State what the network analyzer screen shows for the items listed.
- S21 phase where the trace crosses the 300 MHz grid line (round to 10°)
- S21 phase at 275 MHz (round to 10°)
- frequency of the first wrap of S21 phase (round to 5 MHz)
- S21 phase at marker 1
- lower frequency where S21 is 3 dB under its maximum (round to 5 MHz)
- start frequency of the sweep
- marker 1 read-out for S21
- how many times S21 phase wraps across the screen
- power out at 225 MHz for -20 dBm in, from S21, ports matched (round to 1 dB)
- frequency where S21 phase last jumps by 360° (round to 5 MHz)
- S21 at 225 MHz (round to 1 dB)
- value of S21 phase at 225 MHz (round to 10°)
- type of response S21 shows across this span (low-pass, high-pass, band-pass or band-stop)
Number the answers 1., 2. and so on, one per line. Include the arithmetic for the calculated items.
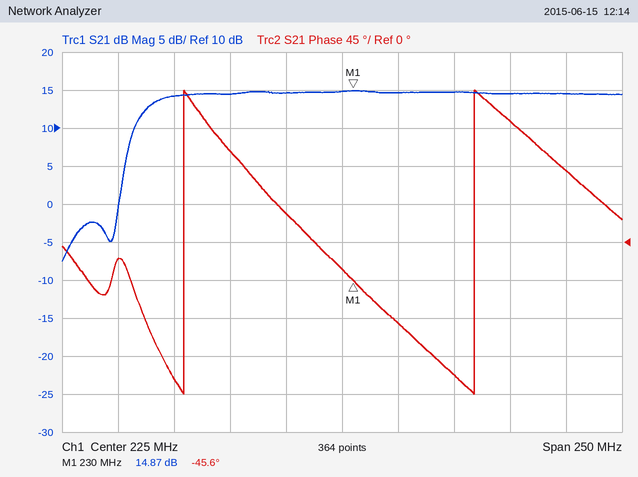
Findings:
1. 140°
2. -160°
3. 155 MHz
4. -45.6°
5. 135 MHz
6. 100 MHz
7. 14.87 dB
8. 2
9. -20 dBm + (15 dB) = -5 dBm
10. 285 MHz
11. 15 dB
12. -30°
13. high-pass
